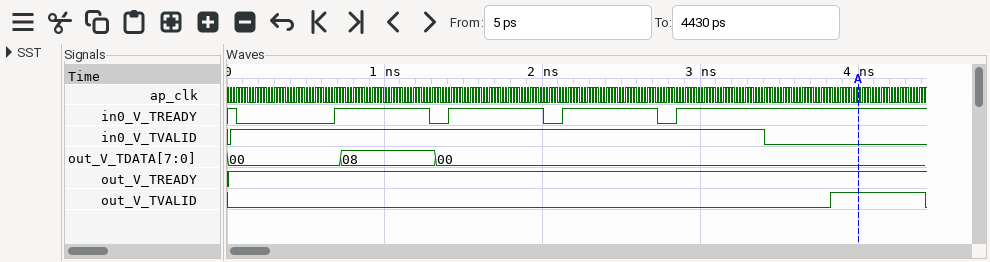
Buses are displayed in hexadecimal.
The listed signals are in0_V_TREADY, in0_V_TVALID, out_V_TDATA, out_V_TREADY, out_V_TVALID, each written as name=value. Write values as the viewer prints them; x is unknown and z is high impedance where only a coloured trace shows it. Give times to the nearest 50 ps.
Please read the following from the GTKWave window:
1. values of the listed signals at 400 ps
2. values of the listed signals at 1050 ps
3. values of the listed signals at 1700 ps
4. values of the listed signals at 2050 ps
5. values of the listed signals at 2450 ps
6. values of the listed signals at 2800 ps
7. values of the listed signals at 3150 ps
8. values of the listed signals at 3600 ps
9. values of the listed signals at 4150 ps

in0_V_TREADY=0, in0_V_TVALID=1, out_V_TDATA=00, out_V_TREADY=1, out_V_TVALID=0
in0_V_TREADY=1, in0_V_TVALID=1, out_V_TDATA=08, out_V_TREADY=1, out_V_TVALID=0
in0_V_TREADY=1, in0_V_TVALID=1, out_V_TDATA=00, out_V_TREADY=1, out_V_TVALID=0
in0_V_TREADY=0, in0_V_TVALID=1, out_V_TDATA=00, out_V_TREADY=1, out_V_TVALID=0
in0_V_TREADY=1, in0_V_TVALID=1, out_V_TDATA=00, out_V_TREADY=1, out_V_TVALID=0
in0_V_TREADY=0, in0_V_TVALID=1, out_V_TDATA=00, out_V_TREADY=1, out_V_TVALID=0
in0_V_TREADY=1, in0_V_TVALID=1, out_V_TDATA=00, out_V_TREADY=1, out_V_TVALID=0
in0_V_TREADY=1, in0_V_TVALID=0, out_V_TDATA=00, out_V_TREADY=1, out_V_TVALID=0
in0_V_TREADY=1, in0_V_TVALID=0, out_V_TDATA=00, out_V_TREADY=1, out_V_TVALID=1
